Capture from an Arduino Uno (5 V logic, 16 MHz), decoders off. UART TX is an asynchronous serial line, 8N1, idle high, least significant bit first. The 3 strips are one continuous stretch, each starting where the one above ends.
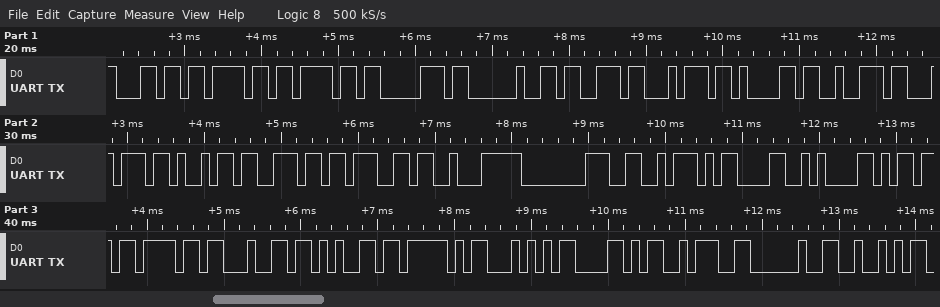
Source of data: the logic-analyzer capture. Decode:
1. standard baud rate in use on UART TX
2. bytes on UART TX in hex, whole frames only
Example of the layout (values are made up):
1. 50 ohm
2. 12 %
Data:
1. 9600 baud
2. 6C 6F 6F 70 20 73 74 61 72 74 69 6E 67 E2 80 A6 0D 0A 6D 6F 64 65 5F 54 58 3A 20 52
